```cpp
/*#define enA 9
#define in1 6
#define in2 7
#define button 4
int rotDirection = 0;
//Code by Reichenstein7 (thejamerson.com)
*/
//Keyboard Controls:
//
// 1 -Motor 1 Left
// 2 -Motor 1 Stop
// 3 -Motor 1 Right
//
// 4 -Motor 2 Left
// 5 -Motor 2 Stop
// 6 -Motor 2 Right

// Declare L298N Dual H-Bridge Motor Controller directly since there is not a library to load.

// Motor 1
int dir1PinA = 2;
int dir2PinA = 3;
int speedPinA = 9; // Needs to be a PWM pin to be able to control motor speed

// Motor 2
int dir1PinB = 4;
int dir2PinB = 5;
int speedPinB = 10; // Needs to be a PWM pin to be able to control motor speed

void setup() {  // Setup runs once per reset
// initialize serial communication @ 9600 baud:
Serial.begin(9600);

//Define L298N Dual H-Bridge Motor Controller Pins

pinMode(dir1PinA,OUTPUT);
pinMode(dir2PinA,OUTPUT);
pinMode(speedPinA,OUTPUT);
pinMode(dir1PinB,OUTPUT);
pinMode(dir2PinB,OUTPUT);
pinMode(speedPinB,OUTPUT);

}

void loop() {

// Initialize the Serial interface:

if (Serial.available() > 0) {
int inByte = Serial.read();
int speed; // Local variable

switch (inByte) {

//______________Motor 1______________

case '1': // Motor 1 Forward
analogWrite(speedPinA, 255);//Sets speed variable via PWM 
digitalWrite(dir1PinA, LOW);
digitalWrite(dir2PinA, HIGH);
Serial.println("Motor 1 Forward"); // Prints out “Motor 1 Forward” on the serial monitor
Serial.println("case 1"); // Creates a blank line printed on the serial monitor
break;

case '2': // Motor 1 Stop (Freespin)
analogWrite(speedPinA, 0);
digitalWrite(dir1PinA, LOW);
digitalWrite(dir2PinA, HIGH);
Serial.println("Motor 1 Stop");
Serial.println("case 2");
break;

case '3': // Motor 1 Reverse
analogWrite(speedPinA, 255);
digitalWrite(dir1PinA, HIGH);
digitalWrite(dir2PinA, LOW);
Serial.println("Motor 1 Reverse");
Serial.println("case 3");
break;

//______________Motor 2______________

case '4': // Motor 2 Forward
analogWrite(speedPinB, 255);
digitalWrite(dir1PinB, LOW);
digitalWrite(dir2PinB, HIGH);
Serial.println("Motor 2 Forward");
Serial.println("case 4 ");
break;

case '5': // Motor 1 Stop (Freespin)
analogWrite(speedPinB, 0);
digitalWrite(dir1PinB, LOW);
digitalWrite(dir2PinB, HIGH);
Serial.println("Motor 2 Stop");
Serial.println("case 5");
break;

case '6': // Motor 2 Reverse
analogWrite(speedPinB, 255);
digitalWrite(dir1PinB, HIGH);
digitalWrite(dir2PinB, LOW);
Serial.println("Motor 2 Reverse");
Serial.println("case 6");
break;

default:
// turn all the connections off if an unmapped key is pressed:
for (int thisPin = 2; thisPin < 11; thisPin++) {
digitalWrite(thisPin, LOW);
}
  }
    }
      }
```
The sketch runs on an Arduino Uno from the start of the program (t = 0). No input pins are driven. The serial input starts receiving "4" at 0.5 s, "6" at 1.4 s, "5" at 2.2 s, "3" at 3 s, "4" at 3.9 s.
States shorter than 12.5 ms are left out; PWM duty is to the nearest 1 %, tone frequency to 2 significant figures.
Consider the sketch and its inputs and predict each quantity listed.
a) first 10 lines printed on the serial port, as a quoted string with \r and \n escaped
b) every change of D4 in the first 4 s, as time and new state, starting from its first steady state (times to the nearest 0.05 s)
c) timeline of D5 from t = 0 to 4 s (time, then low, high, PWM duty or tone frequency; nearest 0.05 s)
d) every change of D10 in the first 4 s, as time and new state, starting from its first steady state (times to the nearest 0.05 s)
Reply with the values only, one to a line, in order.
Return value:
"Motor 2 Forward\r\ncase 4 \r\nMotor 2 Reverse\r\ncase 6\r\nMotor 2 Stop\r\ncase 5\r\nMotor 1 Reverse\r\ncase 3\r\nMotor 2 Forward\r\ncase 4 \r\n"
0 s low; 1.4 s high; 2.2 s low
0 s low; 0.5 s high; 1.4 s low; 2.2 s high
0 s low; 0.5 s high; 2.2 s low; 3.9 s high
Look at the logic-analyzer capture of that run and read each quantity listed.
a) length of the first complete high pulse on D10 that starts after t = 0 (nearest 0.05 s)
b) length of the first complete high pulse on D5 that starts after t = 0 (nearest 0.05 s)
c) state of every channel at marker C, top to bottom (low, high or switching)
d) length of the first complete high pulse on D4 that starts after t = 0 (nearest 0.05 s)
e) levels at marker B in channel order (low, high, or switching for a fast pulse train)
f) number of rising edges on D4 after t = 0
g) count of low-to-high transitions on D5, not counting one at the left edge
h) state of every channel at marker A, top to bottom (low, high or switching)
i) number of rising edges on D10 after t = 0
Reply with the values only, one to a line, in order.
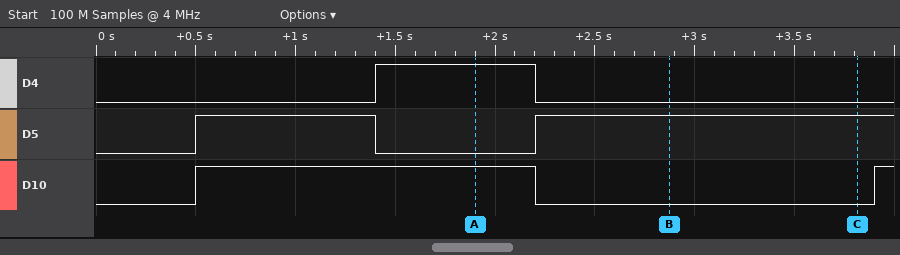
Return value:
1.70 s
0.90 s
D4 low, D5 high, D10 low
0.80 s
D4 low, D5 high, D10 low
1
2
D4 high, D5 low, D10 high
2
